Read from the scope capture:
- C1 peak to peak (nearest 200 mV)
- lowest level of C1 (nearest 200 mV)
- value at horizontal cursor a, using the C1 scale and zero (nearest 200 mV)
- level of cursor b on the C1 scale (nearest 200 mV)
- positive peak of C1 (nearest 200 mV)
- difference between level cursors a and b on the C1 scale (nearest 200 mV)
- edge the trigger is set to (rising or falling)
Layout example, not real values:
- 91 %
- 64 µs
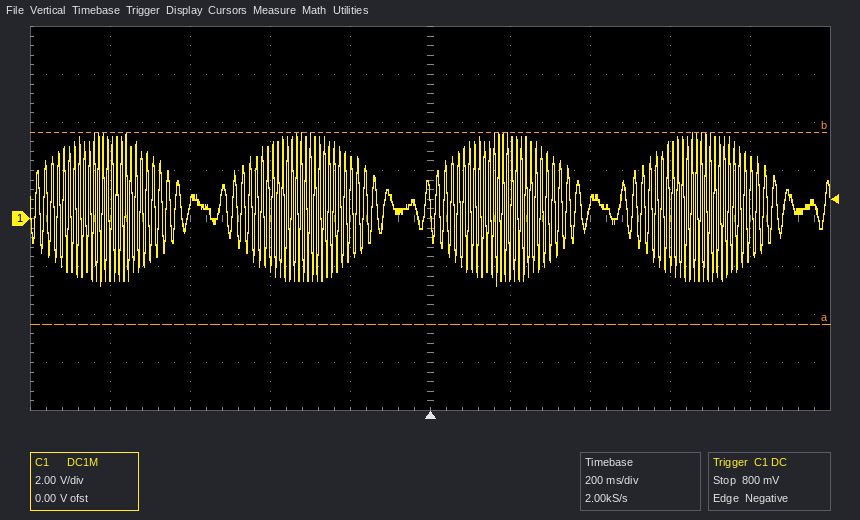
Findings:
- 6.4 V
- -2.8 V
- -4.4 V
- 3.6 V
- 3.6 V
- 8.0 V
- falling
